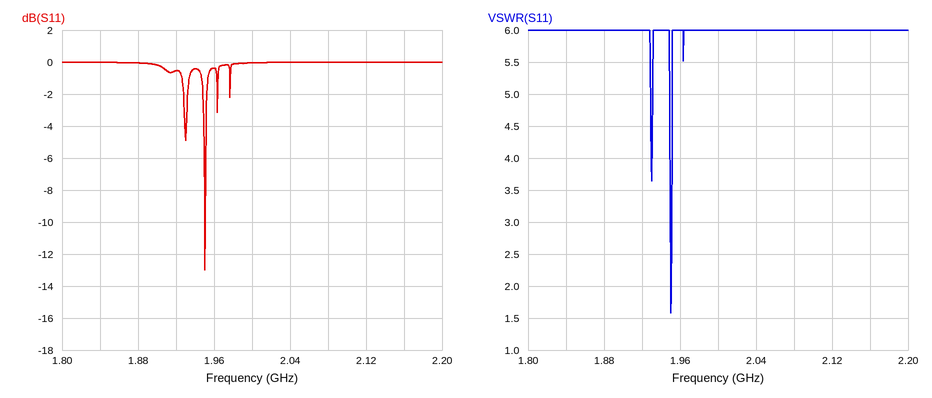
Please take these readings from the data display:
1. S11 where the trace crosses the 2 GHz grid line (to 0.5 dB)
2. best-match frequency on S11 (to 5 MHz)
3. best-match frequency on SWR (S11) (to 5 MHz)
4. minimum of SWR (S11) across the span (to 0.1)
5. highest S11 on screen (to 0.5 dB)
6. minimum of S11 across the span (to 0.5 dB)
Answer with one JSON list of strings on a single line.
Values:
["0.0 dB", "1.950 GHz", "1.950 GHz", "1.6", "0.0 dB", "-13.0 dB"]
